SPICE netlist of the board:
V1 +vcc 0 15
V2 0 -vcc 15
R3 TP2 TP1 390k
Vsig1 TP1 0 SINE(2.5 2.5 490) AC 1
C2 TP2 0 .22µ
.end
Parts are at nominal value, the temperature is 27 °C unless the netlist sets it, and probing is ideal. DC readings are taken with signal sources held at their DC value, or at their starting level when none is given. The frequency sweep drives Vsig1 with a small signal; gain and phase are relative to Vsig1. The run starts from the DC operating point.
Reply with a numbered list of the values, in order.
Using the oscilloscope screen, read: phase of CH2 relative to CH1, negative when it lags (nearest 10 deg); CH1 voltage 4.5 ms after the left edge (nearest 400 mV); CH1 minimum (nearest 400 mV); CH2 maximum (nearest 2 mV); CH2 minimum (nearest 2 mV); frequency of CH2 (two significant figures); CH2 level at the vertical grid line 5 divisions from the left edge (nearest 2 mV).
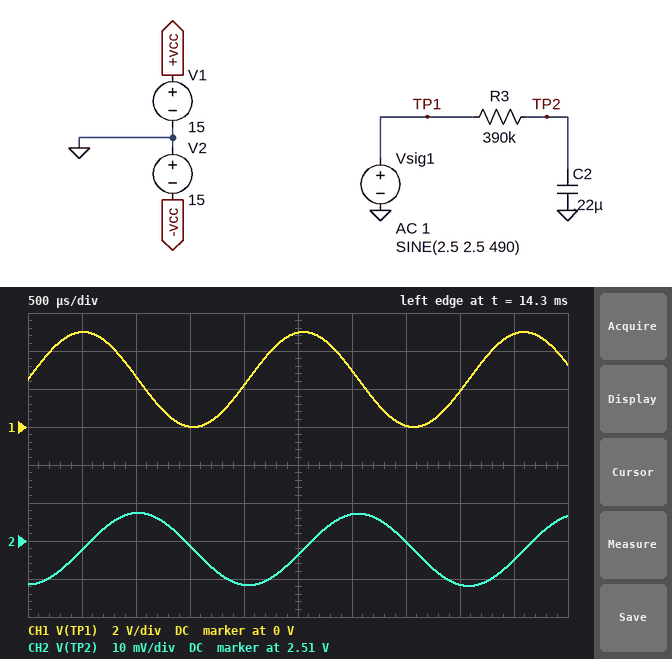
1. -90 deg
2. 4.8 V
3. 0 V
4. 2.518 V
5. 2.498 V
6. 490 Hz
7. 2.506 V
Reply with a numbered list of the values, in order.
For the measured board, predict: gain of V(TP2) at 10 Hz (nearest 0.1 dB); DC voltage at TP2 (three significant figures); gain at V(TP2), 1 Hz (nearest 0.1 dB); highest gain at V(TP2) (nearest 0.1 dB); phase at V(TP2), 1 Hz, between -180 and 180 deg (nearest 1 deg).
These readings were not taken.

1. -14.8 dB
2. 2.50 V
3. -1.1 dB
4. 0 dB
5. -28 deg
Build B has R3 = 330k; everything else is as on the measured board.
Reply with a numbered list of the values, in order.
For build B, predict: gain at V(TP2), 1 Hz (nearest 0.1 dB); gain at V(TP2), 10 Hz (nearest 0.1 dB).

1. -0.8 dB
2. -13.4 dB
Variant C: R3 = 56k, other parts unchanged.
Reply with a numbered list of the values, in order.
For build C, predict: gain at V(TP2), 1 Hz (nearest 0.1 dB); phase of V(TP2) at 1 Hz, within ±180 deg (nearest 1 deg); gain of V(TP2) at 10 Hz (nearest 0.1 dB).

1. 0 dB
2. -4 deg
3. -2.0 dB
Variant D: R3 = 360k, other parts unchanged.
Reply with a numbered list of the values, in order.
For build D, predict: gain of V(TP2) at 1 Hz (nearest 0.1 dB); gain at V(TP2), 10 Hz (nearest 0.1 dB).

1. -1.0 dB
2. -14.1 dB
